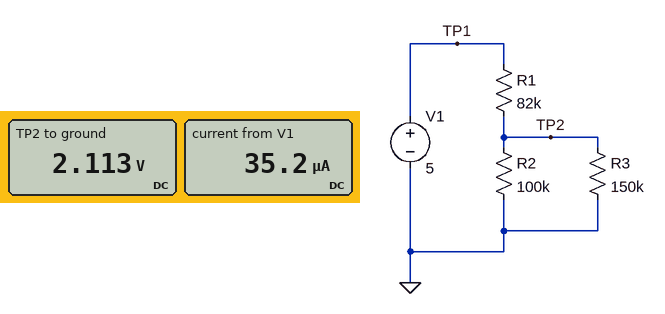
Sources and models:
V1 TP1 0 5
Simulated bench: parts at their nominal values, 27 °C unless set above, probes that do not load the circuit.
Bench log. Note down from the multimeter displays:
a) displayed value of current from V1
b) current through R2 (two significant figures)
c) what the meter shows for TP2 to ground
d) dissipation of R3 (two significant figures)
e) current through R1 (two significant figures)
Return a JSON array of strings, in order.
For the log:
["35.2 µA", "21 µA", "2.113 V", "30 µW", "35 µA"]
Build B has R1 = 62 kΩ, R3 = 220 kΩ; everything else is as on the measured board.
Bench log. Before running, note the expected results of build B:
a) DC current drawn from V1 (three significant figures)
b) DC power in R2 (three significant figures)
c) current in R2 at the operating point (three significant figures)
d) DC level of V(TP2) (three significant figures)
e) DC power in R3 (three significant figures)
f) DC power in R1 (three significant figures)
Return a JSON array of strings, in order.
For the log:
["38.2 µA", "69.1 µW", "26.3 µA", "2.63 V", "31.4 µW", "90.7 µW"]
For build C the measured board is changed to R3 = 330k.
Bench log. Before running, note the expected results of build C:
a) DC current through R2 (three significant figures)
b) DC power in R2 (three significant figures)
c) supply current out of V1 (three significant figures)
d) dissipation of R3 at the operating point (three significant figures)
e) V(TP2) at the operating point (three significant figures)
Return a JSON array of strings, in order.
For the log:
["24.2 µA", "58.4 µW", "31.5 µA", "17.7 µW", "2.42 V"]
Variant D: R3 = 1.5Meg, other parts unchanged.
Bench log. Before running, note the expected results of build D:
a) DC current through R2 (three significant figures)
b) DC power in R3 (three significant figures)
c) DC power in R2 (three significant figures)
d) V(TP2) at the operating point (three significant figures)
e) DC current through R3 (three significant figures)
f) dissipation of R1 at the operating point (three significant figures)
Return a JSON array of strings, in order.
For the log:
["26.7 µA", "4.74 µW", "71.1 µW", "2.67 V", "1.78 µA", "66.4 µW"]
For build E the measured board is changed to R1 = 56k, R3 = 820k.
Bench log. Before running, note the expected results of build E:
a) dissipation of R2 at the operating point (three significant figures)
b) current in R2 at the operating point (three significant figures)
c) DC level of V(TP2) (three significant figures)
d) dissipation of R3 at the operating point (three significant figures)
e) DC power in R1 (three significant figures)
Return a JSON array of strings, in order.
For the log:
["94.3 µW", "30.7 µA", "3.07 V", "11.5 µW", "66.5 µW"]
